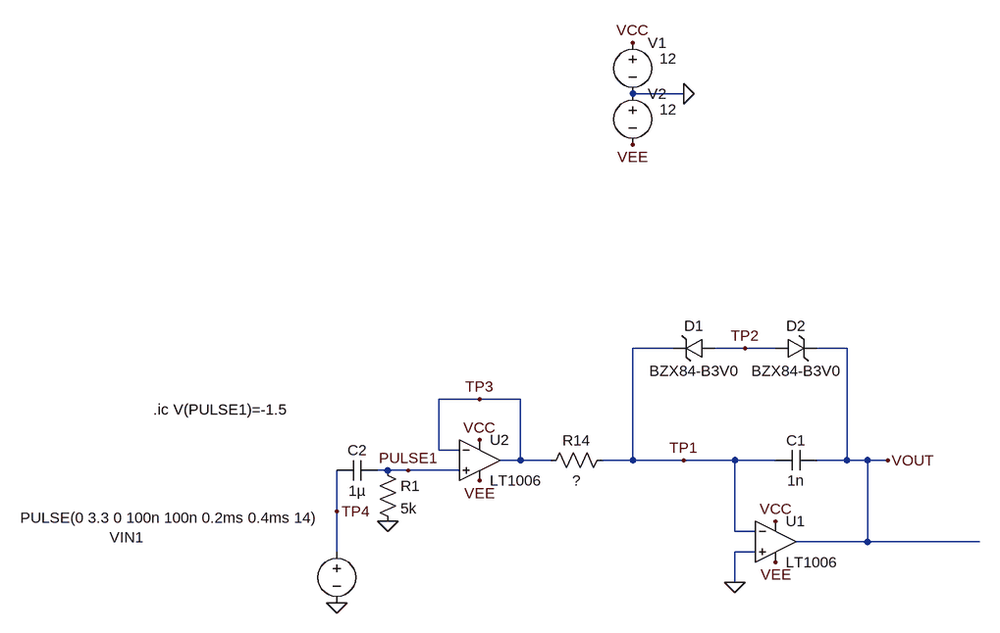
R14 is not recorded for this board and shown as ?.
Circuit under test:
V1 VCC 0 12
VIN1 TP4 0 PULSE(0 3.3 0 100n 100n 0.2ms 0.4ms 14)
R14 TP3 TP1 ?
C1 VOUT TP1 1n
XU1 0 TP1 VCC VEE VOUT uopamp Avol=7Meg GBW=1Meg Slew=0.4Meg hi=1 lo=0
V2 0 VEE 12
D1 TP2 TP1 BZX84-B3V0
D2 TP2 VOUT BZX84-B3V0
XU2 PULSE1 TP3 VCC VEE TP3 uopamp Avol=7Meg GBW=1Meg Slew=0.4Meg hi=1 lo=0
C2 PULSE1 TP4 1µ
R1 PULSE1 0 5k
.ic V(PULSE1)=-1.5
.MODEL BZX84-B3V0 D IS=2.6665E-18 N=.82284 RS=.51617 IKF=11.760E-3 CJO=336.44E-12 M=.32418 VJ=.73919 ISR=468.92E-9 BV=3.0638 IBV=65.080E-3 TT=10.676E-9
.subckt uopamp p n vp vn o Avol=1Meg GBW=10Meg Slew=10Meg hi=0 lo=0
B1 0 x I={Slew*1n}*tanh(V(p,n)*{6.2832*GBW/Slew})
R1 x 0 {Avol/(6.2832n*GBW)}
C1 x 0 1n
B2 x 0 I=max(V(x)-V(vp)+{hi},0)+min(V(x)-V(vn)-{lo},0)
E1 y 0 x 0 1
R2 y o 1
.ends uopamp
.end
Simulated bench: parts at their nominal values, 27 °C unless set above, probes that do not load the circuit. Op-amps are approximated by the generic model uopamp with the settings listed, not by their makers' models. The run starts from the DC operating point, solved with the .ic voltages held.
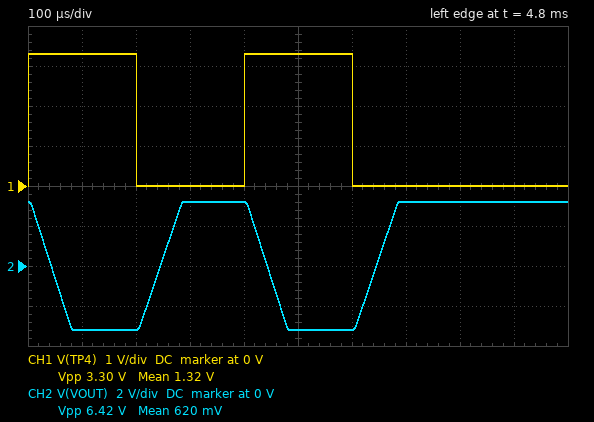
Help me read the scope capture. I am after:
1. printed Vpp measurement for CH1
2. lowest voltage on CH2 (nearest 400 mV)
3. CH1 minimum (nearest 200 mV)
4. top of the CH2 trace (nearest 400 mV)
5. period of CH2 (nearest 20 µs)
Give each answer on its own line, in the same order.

3.30 V
-3.2 V
0 V
3.2 V
400 µs
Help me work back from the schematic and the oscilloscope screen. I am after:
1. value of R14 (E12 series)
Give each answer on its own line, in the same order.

18 kΩ
